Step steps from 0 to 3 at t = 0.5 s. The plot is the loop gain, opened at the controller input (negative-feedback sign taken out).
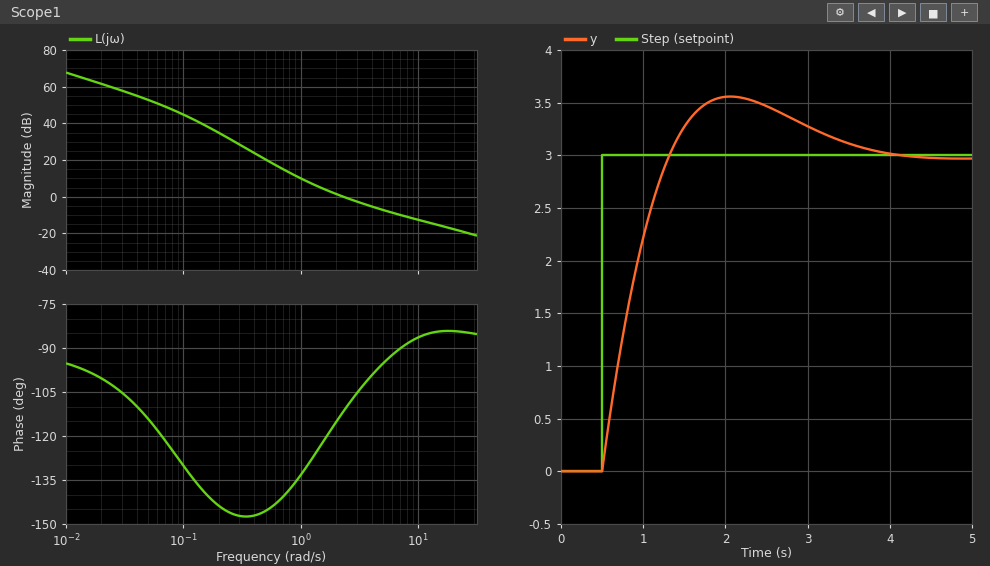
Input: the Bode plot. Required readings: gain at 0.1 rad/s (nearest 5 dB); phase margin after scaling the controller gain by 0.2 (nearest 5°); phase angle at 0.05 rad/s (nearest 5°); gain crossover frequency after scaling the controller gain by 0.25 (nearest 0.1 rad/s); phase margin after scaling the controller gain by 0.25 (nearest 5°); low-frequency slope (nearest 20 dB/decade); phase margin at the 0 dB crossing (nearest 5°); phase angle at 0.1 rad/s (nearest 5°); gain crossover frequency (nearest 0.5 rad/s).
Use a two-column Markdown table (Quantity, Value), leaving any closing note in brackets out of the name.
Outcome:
| Quantity | Value |
|---|---|
| gain at 0.1 rad/s | 45 dB |
| phase margin after scaling the controller gain by 0.2 | 40° |
| phase angle at 0.05 rad/s | -115° |
| gain crossover frequency after scaling the controller gain by 0.25 | 0.9 rad/s |
| phase margin after scaling the controller gain by 0.25 | 45° |
| low-frequency slope | -20 dB/decade |
| phase margin at the 0 dB crossing | 70° |
| phase angle at 0.1 rad/s | -130° |
| gain crossover frequency | 2.5 rad/s |
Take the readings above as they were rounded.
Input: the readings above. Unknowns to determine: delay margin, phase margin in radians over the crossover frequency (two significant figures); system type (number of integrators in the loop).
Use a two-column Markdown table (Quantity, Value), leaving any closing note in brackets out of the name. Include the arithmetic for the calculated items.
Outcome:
| Quantity | Value |
|---|---|
| delay margin, phase margin in radians over the crossover frequency | 70 × π / 180 / 2.5 = 0.49 s |
| system type | 1 |
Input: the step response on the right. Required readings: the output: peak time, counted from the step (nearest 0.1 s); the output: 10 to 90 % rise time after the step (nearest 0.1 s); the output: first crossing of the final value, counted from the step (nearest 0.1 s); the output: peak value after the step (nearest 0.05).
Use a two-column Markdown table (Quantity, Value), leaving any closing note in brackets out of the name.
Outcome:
| Quantity | Value |
|---|---|
| the output: peak time, counted from the step | 1.6 s |
| the output: 10 to 90 % rise time after the step | 0.6 s |
| the output: first crossing of the final value, counted from the step | 0.8 s |
| the output: peak value after the step | 3.55 |
